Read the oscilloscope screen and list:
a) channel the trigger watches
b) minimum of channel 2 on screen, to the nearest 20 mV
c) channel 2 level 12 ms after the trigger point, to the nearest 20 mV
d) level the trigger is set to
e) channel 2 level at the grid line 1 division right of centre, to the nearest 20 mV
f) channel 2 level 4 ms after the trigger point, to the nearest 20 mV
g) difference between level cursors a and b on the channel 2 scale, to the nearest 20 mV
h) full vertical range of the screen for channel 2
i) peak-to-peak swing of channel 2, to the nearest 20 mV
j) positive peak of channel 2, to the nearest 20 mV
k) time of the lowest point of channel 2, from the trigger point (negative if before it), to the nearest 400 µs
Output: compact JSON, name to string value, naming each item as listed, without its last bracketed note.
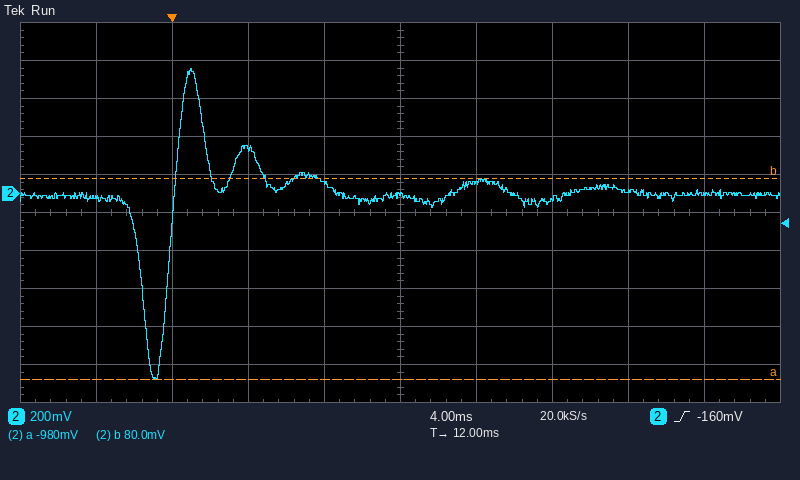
{"channel the trigger watches": "channel 2", "minimum of channel 2 on screen, to the nearest 20 mV": "-980 mV", "channel 2 level 12 ms after the trigger point, to the nearest 20 mV": "-20 mV", "level the trigger is set to": "-160 mV", "channel 2 level at the grid line 1 division right of centre, to the nearest 20 mV": "60 mV", "channel 2 level 4 ms after the trigger point, to the nearest 20 mV": "240 mV", "difference between level cursors a and b on the channel 2 scale, to the nearest 20 mV": "1.06 V", "full vertical range of the screen for channel 2": "2 V", "peak-to-peak swing of channel 2, to the nearest 20 mV": "1.64 V", "positive peak of channel 2, to the nearest 20 mV": "660 mV", "time of the lowest point of channel 2, from the trigger point (negative if before it), to the nearest 400 µs": "-800 µs"}
